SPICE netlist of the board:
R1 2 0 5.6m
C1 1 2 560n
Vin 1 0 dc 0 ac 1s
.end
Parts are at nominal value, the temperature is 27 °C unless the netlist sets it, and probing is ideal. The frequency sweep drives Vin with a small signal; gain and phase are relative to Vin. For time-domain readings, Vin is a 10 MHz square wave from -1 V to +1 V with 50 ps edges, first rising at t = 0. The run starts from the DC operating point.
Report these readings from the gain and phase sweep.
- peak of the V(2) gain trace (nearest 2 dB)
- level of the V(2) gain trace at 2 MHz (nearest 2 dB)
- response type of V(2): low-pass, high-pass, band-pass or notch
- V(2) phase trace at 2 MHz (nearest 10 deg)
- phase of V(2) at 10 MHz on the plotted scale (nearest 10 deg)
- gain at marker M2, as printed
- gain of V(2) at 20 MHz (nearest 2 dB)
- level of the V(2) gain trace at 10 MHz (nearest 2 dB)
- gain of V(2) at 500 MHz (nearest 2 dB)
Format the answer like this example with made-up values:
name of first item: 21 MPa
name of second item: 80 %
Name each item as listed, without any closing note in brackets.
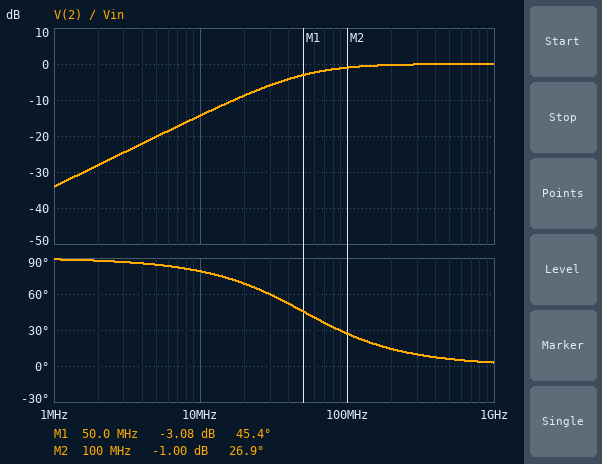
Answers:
peak of the V(2) gain trace: 0 dB
level of the V(2) gain trace at 2 MHz: -28 dB
response type of V(2): low-pass, high-pass, band-pass or notch: high-pass
V(2) phase trace at 2 MHz: 90 deg
phase of V(2) at 10 MHz on the plotted scale: 80 deg
gain at marker M2, as printed: -1.00 dB
gain of V(2) at 20 MHz: -8 dB
level of the V(2) gain trace at 10 MHz: -14 dB
gain of V(2) at 500 MHz: 0 dB
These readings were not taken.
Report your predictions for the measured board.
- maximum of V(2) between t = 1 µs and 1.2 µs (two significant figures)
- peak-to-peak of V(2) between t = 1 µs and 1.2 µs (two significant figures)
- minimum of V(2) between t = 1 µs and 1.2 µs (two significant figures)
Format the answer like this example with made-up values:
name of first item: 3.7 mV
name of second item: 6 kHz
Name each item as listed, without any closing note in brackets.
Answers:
maximum of V(2) between t = 1 µs and 1.2 µs: 2.0 V
peak-to-peak of V(2) between t = 1 µs and 1.2 µs: 4.0 V
minimum of V(2) between t = 1 µs and 1.2 µs: -2.0 V
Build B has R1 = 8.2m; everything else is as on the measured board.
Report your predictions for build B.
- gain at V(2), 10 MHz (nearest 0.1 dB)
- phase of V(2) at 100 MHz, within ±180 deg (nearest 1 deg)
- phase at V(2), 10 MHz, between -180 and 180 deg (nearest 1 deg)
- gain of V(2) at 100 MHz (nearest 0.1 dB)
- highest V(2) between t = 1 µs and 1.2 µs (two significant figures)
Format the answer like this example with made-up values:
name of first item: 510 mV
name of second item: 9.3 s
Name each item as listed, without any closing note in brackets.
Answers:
gain at V(2), 10 MHz: -11.1 dB
phase of V(2) at 100 MHz, within ±180 deg: 19 deg
phase at V(2), 10 MHz, between -180 and 180 deg: 74 deg
gain of V(2) at 100 MHz: -0.5 dB
highest V(2) between t = 1 µs and 1.2 µs: 2.0 V
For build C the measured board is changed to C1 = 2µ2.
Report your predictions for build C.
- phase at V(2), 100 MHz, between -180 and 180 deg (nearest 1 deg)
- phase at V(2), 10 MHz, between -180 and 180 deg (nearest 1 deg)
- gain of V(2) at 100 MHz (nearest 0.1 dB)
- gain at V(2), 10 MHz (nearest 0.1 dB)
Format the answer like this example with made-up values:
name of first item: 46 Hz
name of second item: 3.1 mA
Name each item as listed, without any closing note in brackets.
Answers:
phase at V(2), 100 MHz, between -180 and 180 deg: 7 deg
phase at V(2), 10 MHz, between -180 and 180 deg: 52 deg
gain of V(2) at 100 MHz: -0.1 dB
gain at V(2), 10 MHz: -4.3 dB
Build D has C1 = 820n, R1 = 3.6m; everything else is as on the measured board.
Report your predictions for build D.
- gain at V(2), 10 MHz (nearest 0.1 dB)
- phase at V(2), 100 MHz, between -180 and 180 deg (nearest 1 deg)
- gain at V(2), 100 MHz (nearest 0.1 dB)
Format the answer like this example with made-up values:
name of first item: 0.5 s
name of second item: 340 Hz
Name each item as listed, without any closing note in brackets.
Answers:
gain at V(2), 10 MHz: -14.8 dB
phase at V(2), 100 MHz, between -180 and 180 deg: 28 deg
gain at V(2), 100 MHz: -1.1 dB
